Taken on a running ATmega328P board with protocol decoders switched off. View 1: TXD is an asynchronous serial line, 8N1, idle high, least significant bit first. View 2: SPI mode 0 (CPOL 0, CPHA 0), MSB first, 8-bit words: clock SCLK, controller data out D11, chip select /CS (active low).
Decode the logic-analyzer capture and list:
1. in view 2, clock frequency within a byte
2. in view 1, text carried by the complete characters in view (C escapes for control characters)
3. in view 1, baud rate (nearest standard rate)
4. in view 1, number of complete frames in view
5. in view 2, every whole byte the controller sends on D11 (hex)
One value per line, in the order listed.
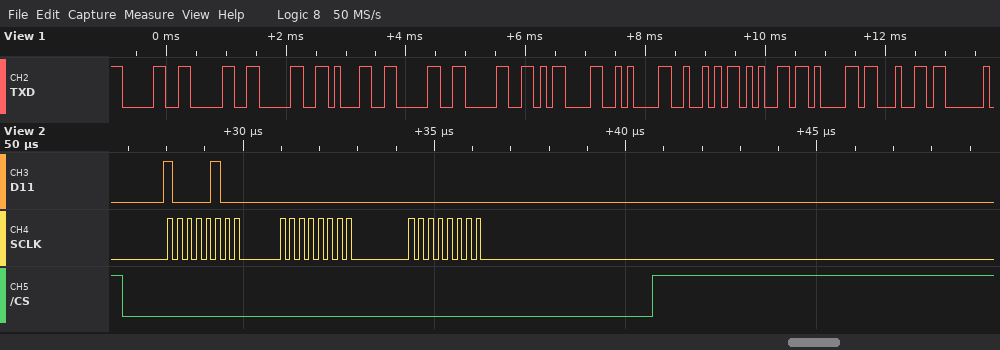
4 MHz
"000100\r\nRead"
9600 baud
12
84 00 00
